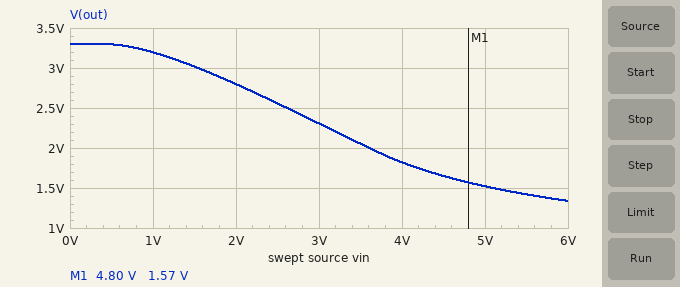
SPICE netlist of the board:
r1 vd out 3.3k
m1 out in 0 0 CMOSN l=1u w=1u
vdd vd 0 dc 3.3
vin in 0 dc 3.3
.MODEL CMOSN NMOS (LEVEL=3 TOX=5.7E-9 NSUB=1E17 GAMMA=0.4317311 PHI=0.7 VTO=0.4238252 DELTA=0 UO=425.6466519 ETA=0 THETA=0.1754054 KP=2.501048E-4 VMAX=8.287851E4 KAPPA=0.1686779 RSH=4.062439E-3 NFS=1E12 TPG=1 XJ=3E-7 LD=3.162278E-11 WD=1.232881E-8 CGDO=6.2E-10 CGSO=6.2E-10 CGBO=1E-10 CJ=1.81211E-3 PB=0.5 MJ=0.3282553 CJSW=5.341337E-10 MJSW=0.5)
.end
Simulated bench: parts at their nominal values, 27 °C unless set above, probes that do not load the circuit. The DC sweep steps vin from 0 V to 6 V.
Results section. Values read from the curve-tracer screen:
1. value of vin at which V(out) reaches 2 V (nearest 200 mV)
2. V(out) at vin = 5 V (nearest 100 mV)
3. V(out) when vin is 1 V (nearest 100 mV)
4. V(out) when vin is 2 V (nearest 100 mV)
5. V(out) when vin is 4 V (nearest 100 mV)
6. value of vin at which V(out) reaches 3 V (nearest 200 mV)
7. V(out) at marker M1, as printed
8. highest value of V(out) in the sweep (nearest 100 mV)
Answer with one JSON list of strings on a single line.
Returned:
["3.6 V", "1.5 V", "3.2 V", "2.8 V", "1.8 V", "1.6 V", "1.57 V", "3.3 V"]
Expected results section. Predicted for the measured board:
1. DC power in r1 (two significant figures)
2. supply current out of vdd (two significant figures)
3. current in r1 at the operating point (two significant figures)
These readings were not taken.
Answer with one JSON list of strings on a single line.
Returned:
["400 µW", "350 µA", "350 µA"]
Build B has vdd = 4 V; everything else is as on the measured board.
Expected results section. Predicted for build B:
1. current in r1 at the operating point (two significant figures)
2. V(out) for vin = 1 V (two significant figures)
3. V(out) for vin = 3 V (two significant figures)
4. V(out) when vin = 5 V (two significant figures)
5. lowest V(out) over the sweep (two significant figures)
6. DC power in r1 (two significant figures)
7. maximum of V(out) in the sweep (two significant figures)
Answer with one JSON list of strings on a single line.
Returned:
["350 µA", "3.9 V", "3.0 V", "2.0 V", "1.7 V", "410 µW", "4.0 V"]
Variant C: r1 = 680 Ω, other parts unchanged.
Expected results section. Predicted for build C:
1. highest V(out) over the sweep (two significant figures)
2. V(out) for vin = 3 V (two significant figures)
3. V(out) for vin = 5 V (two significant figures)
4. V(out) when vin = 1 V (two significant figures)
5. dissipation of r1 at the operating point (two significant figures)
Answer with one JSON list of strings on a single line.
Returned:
["3.3 V", "3.1 V", "2.9 V", "3.3 V", "86 µW"]
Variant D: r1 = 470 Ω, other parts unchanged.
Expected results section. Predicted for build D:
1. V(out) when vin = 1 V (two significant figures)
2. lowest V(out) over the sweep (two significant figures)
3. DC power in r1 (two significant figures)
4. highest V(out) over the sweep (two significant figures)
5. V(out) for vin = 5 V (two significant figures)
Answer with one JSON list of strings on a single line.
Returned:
["3.3 V", "2.9 V", "59 µW", "3.3 V", "3.0 V"]
